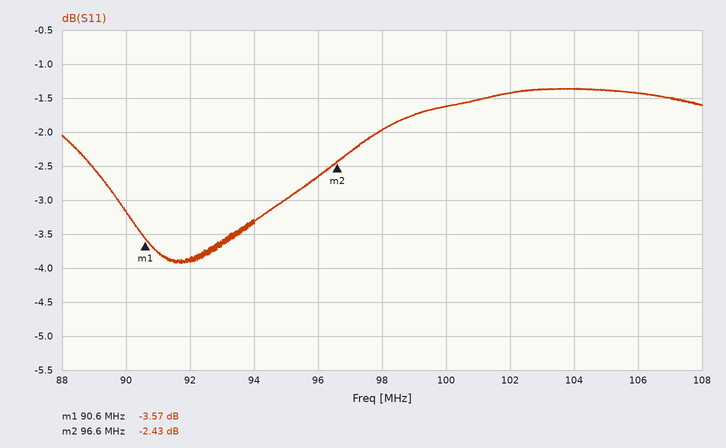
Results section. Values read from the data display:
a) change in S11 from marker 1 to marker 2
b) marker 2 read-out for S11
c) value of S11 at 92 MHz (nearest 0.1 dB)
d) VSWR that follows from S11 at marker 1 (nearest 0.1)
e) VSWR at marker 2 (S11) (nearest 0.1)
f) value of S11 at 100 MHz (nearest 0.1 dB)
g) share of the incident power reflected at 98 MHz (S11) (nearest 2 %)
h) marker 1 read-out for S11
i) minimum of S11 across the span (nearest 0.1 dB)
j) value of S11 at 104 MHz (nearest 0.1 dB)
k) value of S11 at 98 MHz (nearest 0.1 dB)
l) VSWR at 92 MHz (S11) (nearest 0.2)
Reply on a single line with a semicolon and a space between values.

1.14 dB; -2.43 dB; -3.9 dB; 4.9; 7.2; -1.6 dB; 64 %; -3.57 dB; -3.9 dB; -1.4 dB; -2.0 dB; 4.6
